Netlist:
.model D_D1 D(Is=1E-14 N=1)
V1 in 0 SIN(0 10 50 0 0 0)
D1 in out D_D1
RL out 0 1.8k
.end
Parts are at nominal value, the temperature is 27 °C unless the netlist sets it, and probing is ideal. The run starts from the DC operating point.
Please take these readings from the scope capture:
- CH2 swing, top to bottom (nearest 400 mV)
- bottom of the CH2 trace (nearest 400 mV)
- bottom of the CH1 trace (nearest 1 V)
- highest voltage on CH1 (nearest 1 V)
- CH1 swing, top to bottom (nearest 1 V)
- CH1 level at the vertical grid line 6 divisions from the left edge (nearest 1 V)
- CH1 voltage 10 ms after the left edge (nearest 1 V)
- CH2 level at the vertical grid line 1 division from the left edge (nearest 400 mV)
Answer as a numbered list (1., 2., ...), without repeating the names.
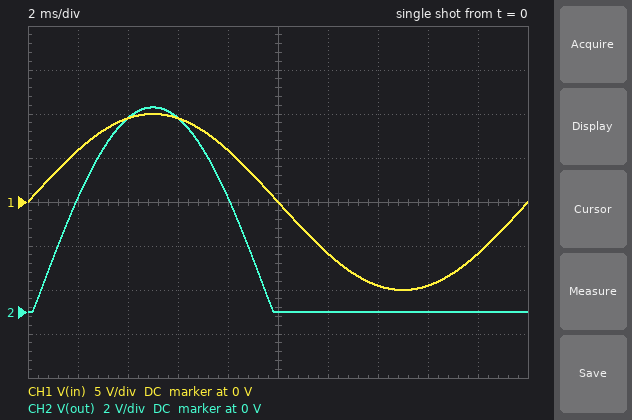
1. 9.2 V
2. 0 V
3. -10 V
4. 10 V
5. 20 V
6. -6 V
7. 0 V
8. 5.2 V
